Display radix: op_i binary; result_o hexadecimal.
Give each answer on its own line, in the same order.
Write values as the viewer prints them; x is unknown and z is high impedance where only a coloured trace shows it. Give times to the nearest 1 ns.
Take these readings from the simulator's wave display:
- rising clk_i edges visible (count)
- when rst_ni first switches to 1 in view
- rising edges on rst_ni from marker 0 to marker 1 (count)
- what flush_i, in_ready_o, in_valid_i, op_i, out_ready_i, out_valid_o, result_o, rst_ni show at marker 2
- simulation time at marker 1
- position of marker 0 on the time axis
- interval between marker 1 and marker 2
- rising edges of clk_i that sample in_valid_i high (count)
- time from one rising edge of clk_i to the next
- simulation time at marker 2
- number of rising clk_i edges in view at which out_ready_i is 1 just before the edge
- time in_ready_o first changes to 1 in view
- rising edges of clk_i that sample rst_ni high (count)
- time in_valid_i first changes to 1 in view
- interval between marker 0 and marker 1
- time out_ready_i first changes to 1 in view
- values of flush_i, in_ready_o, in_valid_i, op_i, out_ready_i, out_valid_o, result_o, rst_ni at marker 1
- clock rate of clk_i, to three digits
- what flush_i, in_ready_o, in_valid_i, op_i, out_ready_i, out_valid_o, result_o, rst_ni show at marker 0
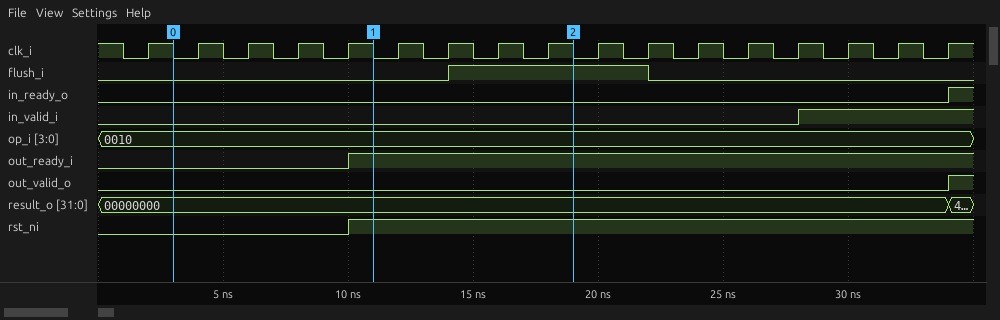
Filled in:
17
10 ns
1
flush_i=1, in_ready_o=0, in_valid_i=0, op_i=0010, out_ready_i=1, out_valid_o=0, result_o=00000000, rst_ni=1
11 ns
3 ns
8 ns
3
2 ns
19 ns
12
34 ns
12
28 ns
8 ns
10 ns
flush_i=0, in_ready_o=0, in_valid_i=0, op_i=0010, out_ready_i=1, out_valid_o=0, result_o=00000000, rst_ni=1
500 MHz
flush_i=0, in_ready_o=0, in_valid_i=0, op_i=0010, out_ready_i=0, out_valid_o=0, result_o=00000000, rst_ni=0
